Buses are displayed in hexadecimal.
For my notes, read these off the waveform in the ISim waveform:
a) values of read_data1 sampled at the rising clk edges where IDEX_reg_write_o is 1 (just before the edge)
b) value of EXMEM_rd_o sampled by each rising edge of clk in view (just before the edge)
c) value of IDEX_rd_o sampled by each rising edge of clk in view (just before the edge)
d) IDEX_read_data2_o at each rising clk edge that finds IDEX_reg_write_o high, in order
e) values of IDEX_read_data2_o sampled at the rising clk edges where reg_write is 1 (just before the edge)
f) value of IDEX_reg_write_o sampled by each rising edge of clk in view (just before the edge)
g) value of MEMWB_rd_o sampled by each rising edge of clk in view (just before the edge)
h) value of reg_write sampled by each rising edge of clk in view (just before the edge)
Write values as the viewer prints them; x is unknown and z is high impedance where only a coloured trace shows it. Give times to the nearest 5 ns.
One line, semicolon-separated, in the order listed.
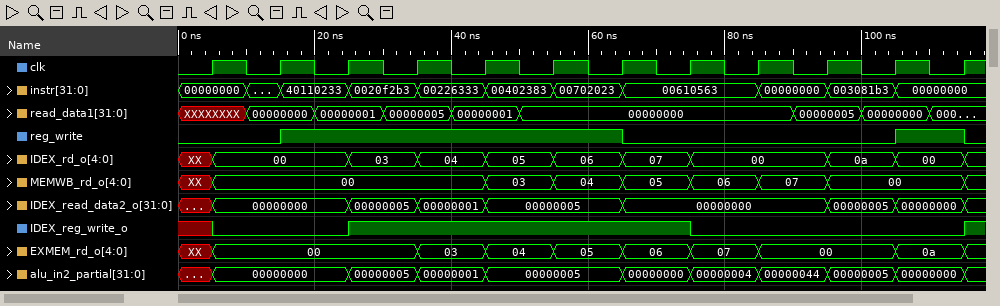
00000005, 00000001, 00000000, 00000000, 00000000; XX, 00, 00, 00, 03, 04, 05, 06, 07, 00, 00, 0a; XX, 00, 00, 03, 04, 05, 06, 07, 00, 00, 0a, 00; 00000005, 00000001, 00000005, 00000005, 00000000; 00000000, 00000005, 00000001, 00000005, 00000005, 00000000; x 0 0 1 1 1 1 1 0 0 0 0; XX, 00, 00, 00, 00, 03, 04, 05, 06, 07, 00, 00; 0 0 1 1 1 1 1 0 0 0 0 1
